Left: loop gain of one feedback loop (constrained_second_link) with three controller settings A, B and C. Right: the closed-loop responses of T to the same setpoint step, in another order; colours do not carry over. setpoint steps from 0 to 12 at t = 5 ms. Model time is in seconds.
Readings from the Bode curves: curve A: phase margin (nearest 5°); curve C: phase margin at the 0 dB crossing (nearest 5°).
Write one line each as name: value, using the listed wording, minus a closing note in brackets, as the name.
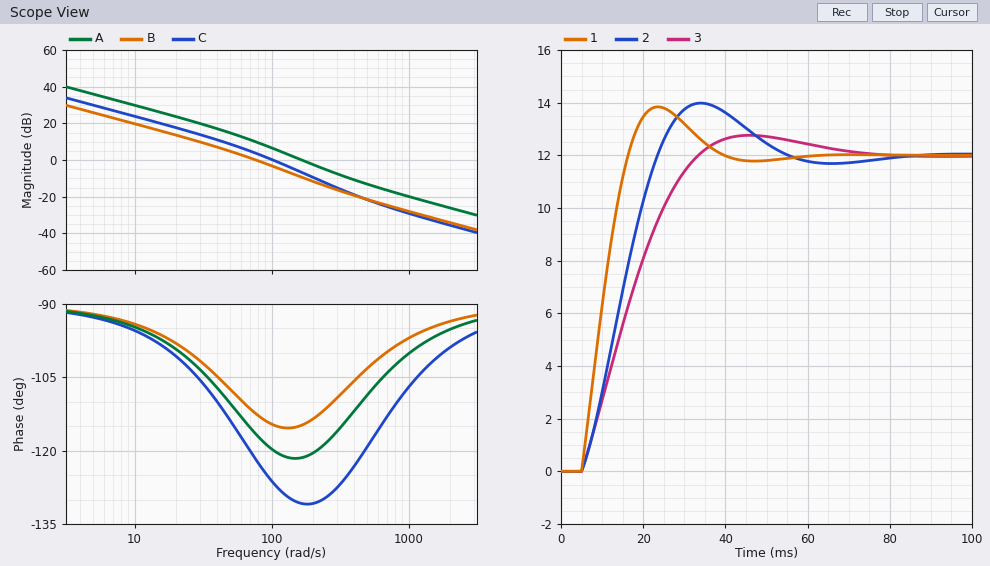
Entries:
curve A: phase margin: 60°
curve C: phase margin at the 0 dB crossing: 55°
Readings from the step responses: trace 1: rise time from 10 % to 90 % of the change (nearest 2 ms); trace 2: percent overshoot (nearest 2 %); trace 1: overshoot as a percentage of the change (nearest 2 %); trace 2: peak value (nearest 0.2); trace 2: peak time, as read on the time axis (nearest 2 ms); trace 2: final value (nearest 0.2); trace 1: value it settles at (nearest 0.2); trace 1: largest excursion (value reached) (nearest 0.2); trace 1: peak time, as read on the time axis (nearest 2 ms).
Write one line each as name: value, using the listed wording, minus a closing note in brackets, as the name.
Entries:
trace 1: rise time from 10 % to 90 % of the change: 8 ms
trace 2: percent overshoot: 16 %
trace 1: overshoot as a percentage of the change: 16 %
trace 2: peak value: 14.0
trace 2: peak time, as read on the time axis: 34 ms
trace 2: final value: 12.0
trace 1: value it settles at: 12.0
trace 1: largest excursion (value reached): 13.8
trace 1: peak time, as read on the time axis: 24 ms
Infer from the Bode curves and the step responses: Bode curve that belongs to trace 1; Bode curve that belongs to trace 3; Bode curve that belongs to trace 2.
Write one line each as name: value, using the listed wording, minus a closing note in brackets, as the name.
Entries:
Bode curve that belongs to trace 1: A
Bode curve that belongs to trace 3: B
Bode curve that belongs to trace 2: C
